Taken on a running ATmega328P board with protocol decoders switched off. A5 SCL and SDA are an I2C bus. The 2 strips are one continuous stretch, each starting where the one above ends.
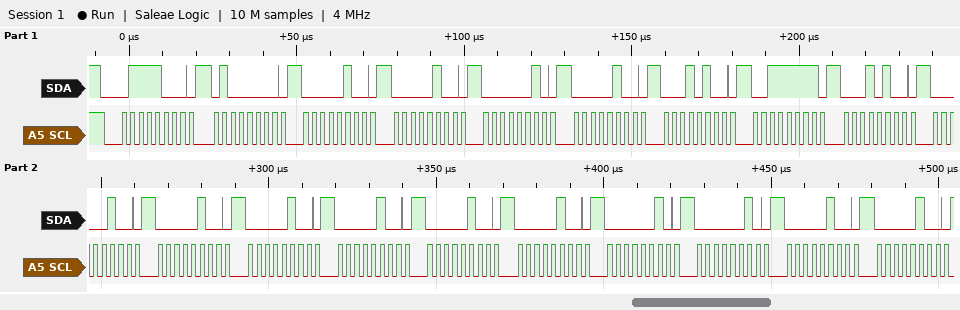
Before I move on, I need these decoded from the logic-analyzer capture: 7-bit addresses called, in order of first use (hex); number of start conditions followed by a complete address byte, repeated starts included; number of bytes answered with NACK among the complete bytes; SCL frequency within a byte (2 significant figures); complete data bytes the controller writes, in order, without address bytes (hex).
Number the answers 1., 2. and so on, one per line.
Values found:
1. 0x3C
2. 1
3. 0
4. 400 kHz
5. 40 04 04 02 04 14 3F 14 04 04 04 04 04 04 02 02 04 04
